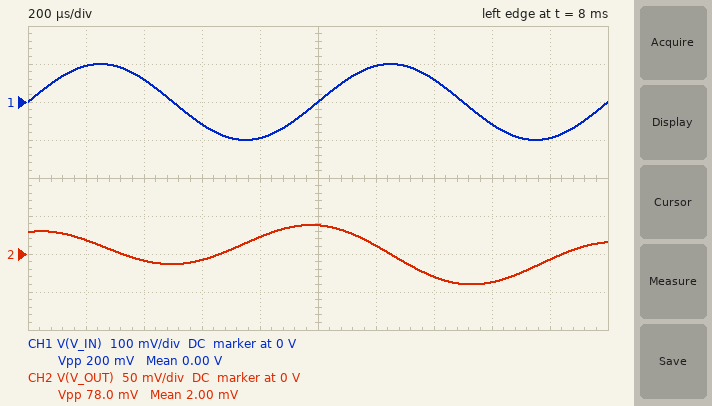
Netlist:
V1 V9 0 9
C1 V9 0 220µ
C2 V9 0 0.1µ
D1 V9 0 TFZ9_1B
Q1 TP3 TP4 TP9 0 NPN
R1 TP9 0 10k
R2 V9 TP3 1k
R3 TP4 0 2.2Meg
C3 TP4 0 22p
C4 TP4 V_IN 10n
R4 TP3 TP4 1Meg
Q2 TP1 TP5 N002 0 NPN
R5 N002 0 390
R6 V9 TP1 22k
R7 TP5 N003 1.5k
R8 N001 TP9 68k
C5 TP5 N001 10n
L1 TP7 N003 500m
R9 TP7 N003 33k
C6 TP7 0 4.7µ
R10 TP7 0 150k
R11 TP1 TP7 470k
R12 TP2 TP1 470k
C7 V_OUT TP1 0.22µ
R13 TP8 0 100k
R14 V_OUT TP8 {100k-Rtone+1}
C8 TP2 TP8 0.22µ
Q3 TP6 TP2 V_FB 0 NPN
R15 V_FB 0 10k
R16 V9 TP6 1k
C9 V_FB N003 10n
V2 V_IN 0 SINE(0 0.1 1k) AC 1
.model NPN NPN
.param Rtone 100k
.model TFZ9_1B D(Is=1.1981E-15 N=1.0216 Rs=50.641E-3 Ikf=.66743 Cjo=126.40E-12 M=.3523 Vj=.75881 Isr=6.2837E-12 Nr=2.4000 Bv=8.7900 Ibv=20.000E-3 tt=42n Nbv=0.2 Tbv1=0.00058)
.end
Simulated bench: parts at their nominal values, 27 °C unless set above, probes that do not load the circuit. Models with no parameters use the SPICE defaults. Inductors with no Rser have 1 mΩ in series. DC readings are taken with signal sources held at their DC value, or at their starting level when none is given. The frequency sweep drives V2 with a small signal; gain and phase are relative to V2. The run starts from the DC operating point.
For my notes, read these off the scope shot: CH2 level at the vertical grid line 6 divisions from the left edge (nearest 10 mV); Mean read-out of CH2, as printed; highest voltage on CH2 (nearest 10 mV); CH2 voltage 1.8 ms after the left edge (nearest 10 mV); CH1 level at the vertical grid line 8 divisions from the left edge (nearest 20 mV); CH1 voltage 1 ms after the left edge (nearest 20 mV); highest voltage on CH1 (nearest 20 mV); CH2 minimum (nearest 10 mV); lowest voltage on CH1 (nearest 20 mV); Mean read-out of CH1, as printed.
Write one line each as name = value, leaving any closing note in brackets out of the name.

CH2 level at the vertical grid line 6 divisions from the left edge = 10 mV
Mean read-out of CH2, as printed = 2.00 mV
highest voltage on CH2 = 40 mV
CH2 voltage 1.8 ms after the left edge = -10 mV
CH1 level at the vertical grid line 8 divisions from the left edge = -60 mV
CH1 voltage 1 ms after the left edge = 0 V
highest voltage on CH1 = 100 mV
CH2 minimum = -40 mV
lowest voltage on CH1 = -100 mV
Mean read-out of CH1, as printed = 0.00 V
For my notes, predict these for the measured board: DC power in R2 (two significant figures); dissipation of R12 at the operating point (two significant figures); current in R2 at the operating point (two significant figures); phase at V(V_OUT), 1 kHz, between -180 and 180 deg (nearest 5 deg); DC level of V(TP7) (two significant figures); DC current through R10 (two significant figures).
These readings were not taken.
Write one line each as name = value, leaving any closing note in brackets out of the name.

DC power in R2 = 98 µW
dissipation of R12 at the operating point = 2.8 µW
current in R2 at the operating point = 310 µA
phase at V(V_OUT), 1 kHz, between -180 and 180 deg = 90 deg
DC level of V(TP7) = 820 mV
DC current through R10 = 5.4 µA
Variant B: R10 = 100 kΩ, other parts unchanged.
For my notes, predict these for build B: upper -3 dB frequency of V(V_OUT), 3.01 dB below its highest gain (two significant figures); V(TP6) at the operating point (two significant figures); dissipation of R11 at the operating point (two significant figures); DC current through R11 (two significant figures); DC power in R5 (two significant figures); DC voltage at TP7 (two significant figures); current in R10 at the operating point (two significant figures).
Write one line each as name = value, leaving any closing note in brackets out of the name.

upper -3 dB frequency of V(V_OUT), 3.01 dB below its highest gain = 440 Hz
V(TP6) at the operating point = 8.7 V
dissipation of R11 at the operating point = 42 µW
DC current through R11 = 9.5 µA
DC power in R5 = 9.9 µW
DC voltage at TP7 = 790 mV
current in R10 at the operating point = 7.9 µA
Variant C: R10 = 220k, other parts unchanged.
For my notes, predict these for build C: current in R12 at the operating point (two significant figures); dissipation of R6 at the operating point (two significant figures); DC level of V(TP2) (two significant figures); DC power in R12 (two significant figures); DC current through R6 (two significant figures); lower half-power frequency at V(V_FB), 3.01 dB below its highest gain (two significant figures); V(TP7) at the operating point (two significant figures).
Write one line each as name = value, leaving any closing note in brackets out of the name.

current in R12 at the operating point = 2.0 µA
dissipation of R6 at the operating point = 1.3 mW
DC level of V(TP2) = 2.8 V
DC power in R12 = 1.9 µW
DC current through R6 = 240 µA
lower half-power frequency at V(V_FB), 3.01 dB below its highest gain = 390 Hz
V(TP7) at the operating point = 830 mV
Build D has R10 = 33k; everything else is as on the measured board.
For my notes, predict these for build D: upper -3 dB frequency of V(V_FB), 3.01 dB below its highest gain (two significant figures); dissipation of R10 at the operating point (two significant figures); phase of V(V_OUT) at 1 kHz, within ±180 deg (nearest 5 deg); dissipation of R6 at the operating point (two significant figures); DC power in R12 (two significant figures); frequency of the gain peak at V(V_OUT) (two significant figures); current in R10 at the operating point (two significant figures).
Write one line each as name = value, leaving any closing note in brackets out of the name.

upper -3 dB frequency of V(V_FB), 3.01 dB below its highest gain = 2.4 kHz
dissipation of R10 at the operating point = 9.4 µW
phase of V(V_OUT) at 1 kHz, within ±180 deg = -110 deg
dissipation of R6 at the operating point = 11 µW
DC power in R12 = 13 µW
frequency of the gain peak at V(V_OUT) = 2.1 kHz
current in R10 at the operating point = 17 µA
